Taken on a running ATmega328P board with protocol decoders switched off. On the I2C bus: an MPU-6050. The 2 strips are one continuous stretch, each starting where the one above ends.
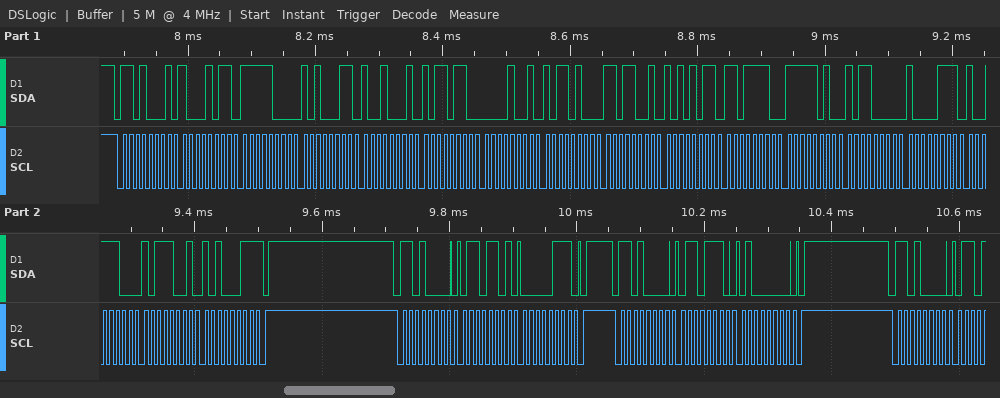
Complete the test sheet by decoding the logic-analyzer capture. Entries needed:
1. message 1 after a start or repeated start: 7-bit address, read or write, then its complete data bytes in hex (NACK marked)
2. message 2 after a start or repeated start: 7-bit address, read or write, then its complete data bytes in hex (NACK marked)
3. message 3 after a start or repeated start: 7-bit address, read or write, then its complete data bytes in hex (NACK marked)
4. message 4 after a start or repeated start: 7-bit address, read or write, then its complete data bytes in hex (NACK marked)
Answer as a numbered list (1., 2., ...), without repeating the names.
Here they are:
1. 0x68 read: 8B F8 A3 91 B6 09 B4 D9 AB DE FA B0 87 9C B9 A3 NACK
2. 0x68 write: 6D 07
3. 0x68 write: 6E 40
4. 0x68 write
